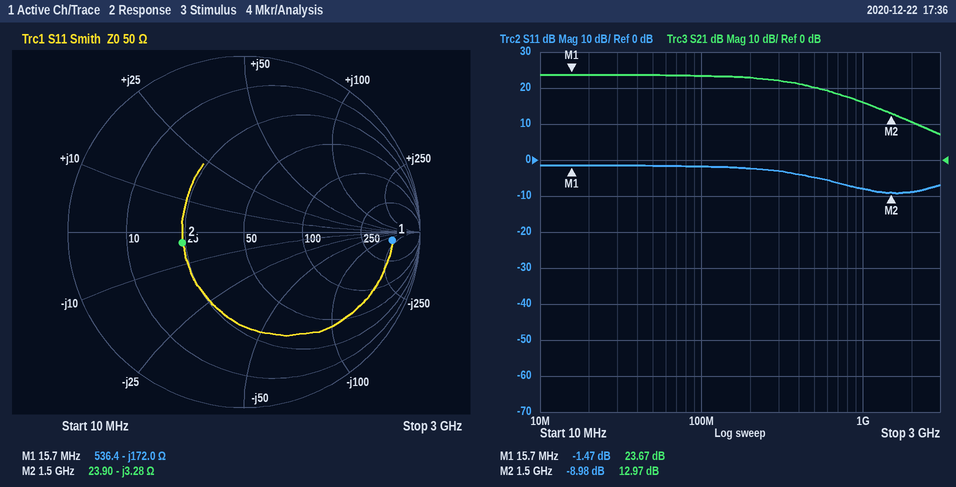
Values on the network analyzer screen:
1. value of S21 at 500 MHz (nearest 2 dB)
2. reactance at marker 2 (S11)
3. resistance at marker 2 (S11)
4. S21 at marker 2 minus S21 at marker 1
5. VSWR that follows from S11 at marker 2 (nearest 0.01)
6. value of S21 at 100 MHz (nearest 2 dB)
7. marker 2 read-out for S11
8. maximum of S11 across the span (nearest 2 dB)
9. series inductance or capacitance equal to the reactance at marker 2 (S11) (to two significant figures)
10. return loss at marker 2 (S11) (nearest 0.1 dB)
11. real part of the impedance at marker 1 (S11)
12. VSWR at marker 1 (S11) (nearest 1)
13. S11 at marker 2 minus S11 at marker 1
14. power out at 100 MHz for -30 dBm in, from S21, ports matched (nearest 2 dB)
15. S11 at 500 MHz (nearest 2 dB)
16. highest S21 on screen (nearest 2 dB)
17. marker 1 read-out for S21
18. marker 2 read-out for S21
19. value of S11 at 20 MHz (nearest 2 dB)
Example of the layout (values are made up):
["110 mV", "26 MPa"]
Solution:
["20 dB", "-3.28 Ω", "23.90 Ω", "-10.70 dB", "2.10", "24 dB", "-8.98 dB", "-2 dB", "32 pF", "9.0 dB", "536.4 Ω", "12", "-7.51 dB", "-6 dBm", "-4 dB", "24 dB", "23.67 dB", "12.97 dB", "-2 dB"]
